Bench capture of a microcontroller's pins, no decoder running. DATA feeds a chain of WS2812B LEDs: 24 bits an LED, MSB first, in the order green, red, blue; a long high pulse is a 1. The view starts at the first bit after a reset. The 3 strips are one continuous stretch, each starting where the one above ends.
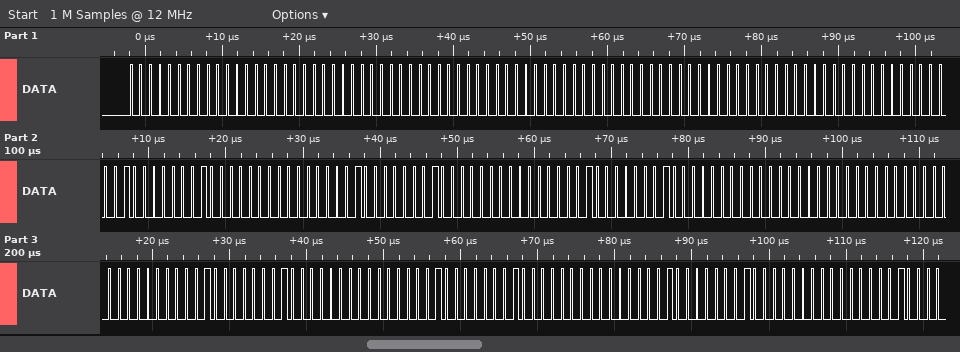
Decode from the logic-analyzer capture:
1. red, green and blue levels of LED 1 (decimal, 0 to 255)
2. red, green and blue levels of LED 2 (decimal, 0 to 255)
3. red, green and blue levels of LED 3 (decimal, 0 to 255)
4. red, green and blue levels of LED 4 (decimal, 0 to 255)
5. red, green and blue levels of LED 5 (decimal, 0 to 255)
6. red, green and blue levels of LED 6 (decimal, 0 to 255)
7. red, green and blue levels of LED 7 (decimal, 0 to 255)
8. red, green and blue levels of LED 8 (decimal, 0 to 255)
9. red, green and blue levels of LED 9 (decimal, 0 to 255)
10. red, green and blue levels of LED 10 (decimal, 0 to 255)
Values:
0, 0, 0
0, 0, 0
0, 0, 0
1, 0, 1
1, 0, 1
1, 0, 1
0, 0, 0
1, 0, 1
1, 0, 1
1, 0, 1
